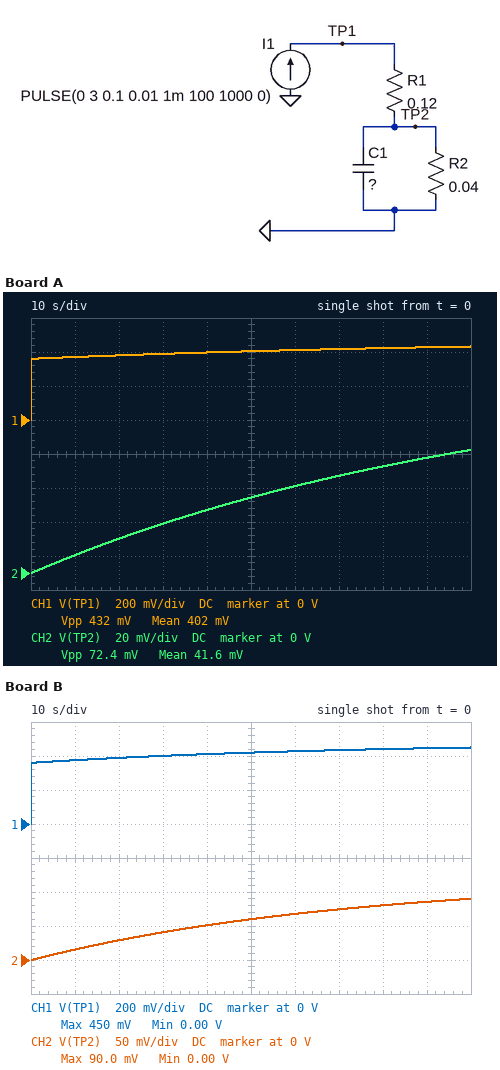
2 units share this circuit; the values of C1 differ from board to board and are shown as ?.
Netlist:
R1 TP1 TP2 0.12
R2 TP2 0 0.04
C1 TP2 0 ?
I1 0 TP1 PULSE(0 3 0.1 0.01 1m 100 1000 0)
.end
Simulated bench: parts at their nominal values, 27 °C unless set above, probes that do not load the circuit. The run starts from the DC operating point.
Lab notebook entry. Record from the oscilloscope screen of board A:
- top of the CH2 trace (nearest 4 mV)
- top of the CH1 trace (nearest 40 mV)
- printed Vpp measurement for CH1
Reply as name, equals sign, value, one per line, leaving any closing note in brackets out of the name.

top of the CH2 trace = 72 mV
top of the CH1 trace = 440 mV
printed Vpp measurement for CH1 = 432 mV
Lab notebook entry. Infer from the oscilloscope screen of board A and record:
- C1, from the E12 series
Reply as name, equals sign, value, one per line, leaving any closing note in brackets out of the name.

C1, from the E12 series = 2.7 kF
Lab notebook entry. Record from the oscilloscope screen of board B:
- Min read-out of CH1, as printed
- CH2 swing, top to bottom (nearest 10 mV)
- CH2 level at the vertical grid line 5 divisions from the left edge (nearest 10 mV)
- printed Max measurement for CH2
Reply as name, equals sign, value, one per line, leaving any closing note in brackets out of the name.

Min read-out of CH1, as printed = 0.00 V
CH2 swing, top to bottom = 90 mV
CH2 level at the vertical grid line 5 divisions from the left edge = 60 mV
printed Max measurement for CH2 = 90.0 mV
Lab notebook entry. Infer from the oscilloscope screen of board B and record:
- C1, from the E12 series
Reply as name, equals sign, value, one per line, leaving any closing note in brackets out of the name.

C1, from the E12 series = 1.8 kF
